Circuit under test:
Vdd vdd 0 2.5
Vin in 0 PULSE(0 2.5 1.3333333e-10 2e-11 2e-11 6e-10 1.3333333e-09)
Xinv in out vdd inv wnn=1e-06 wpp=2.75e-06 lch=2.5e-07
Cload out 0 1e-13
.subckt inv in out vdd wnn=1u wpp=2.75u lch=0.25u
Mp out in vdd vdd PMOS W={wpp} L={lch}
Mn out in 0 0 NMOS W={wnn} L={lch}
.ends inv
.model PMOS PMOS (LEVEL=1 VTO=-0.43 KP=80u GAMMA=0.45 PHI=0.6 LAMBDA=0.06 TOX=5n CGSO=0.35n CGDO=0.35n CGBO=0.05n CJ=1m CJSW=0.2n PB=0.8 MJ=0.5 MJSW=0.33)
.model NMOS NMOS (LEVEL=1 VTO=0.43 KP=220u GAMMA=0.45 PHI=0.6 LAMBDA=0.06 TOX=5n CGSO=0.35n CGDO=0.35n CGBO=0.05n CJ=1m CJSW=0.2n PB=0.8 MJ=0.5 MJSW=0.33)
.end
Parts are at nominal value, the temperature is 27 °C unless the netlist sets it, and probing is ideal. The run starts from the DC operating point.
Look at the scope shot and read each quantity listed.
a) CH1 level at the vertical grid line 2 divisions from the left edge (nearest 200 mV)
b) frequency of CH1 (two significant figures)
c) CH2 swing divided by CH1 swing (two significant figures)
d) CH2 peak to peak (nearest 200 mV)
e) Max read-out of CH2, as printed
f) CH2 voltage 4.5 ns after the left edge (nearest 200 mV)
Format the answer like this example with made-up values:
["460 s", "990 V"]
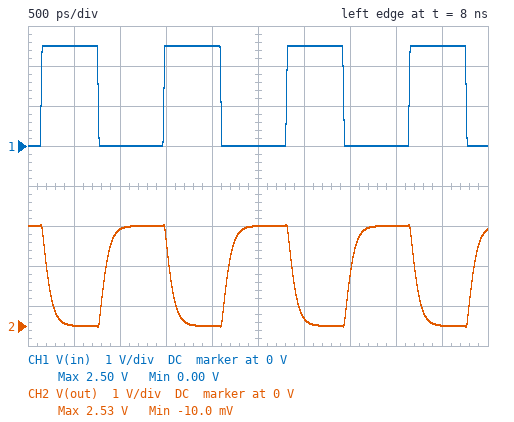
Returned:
["0 V", "750 MHz", "1.0", "2.6 V", "2.53 V", "0 V"]
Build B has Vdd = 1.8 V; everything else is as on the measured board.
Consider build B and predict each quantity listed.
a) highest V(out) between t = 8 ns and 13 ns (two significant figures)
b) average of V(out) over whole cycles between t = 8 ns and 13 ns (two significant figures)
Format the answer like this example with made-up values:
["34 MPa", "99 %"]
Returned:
["1.8 V", "880 mV"]
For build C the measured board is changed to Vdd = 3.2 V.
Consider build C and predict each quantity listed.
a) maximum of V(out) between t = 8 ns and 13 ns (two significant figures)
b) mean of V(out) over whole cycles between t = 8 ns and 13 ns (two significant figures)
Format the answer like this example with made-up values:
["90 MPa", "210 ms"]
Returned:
["3.2 V", "1.8 V"]
